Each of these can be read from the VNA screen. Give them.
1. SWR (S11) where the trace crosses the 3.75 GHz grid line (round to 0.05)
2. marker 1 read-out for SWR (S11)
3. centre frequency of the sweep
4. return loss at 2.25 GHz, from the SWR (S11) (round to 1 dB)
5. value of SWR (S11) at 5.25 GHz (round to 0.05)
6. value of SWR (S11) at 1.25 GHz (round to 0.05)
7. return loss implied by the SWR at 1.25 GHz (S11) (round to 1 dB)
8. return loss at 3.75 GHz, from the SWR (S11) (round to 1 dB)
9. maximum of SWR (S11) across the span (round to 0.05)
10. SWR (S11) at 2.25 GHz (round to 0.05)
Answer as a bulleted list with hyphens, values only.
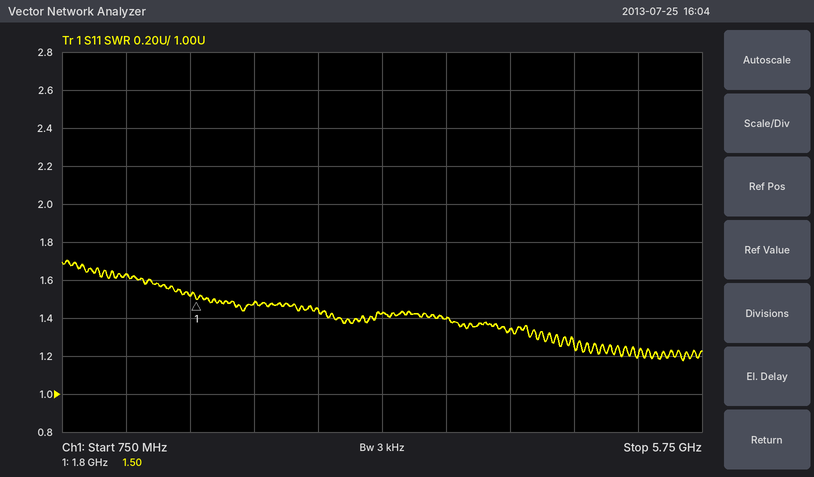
- 1.40
- 1.50
- 3.25 GHz
- 14 dB
- 1.20
- 1.65
- 12 dB
- 16 dB
- 1.70
- 1.50
